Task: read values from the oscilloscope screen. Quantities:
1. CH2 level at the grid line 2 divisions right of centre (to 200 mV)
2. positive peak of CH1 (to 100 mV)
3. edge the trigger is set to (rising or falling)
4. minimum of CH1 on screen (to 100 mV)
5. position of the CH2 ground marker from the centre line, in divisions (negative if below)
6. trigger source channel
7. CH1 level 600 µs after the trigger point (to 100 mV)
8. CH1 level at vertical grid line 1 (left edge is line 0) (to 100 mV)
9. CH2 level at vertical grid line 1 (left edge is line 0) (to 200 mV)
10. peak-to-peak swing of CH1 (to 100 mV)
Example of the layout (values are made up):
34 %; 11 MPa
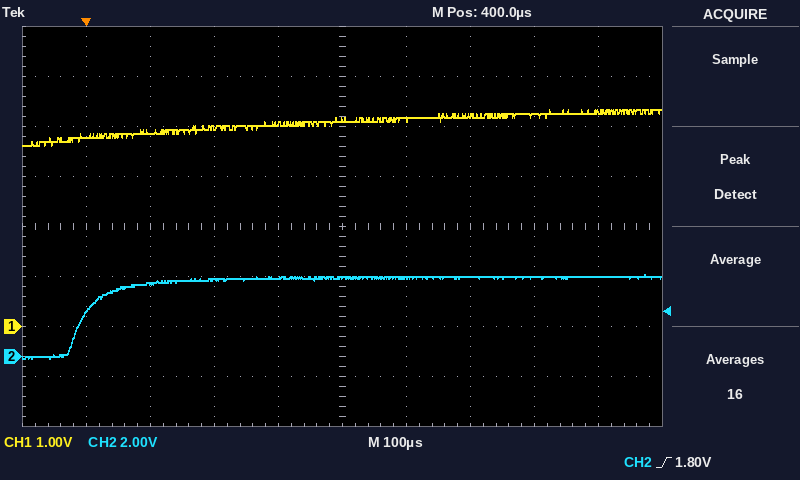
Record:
3.2 V; 4.3 V; rising; 3.6 V; -2.6 div; CH2; 4.2 V; 3.8 V; 1.8 V; 700 mV
